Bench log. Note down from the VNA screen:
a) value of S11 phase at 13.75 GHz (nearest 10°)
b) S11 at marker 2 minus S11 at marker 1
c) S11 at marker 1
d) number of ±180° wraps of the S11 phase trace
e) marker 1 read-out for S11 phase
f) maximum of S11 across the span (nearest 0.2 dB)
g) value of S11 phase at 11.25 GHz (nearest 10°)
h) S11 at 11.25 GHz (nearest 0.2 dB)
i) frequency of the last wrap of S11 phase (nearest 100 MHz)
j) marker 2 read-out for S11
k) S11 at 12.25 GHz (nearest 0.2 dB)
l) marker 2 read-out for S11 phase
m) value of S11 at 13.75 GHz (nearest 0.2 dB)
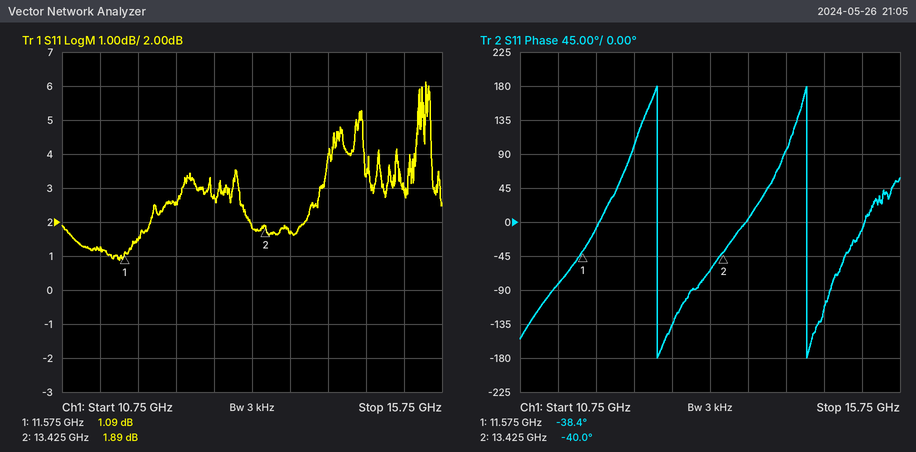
0°
0.80 dB
1.09 dB
2
-38.4°
6.2 dB
-80°
1.2 dB
14.5 GHz
1.89 dB
2.6 dB
-40.0°
1.6 dB
